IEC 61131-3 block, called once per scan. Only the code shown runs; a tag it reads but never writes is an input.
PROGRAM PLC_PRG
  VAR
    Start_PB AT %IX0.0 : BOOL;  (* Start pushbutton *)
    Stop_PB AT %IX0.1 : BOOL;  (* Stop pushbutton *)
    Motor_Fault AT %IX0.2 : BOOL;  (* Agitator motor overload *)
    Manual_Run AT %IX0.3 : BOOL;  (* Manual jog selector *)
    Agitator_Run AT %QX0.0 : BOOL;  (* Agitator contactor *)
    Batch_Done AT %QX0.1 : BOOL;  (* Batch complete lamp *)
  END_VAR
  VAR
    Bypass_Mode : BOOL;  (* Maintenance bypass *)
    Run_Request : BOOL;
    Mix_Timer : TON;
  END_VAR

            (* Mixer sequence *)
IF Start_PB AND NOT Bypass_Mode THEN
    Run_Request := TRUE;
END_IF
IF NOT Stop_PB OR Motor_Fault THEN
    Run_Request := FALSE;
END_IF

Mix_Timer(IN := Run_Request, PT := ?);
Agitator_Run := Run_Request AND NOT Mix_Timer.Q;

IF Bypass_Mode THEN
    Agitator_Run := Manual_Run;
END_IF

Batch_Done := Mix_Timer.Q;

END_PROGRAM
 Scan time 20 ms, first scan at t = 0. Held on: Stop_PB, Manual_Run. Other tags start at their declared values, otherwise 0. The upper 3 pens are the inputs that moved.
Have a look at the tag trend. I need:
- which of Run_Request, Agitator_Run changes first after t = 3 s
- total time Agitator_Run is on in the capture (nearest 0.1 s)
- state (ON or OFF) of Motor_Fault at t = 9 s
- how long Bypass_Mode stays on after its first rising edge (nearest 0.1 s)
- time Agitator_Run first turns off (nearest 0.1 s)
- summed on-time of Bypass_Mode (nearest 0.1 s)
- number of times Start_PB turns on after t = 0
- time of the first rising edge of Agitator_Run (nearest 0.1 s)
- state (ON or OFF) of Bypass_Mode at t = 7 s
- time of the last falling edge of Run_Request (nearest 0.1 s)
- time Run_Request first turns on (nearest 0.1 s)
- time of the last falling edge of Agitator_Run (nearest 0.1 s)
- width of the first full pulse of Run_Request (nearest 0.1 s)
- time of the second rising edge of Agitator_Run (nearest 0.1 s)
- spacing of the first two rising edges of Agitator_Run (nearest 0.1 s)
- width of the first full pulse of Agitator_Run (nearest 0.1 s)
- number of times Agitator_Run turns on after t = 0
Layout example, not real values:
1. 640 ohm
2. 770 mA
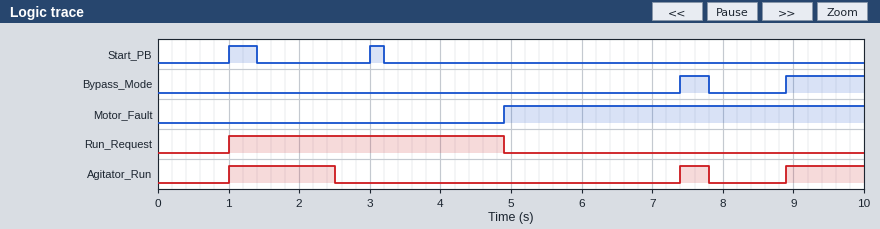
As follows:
1. Run_Request
2. 3.0 s
3. ON
4. 0.4 s
5. 2.5 s
6. 1.5 s
7. 2
8. 1.0 s
9. OFF
10. 4.9 s
11. 1.0 s
12. 7.8 s
13. 3.9 s
14. 7.4 s
15. 6.4 s
16. 1.5 s
17. 3
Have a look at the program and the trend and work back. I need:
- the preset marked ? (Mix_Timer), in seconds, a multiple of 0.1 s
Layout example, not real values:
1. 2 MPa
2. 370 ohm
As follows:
1. 1.5 s
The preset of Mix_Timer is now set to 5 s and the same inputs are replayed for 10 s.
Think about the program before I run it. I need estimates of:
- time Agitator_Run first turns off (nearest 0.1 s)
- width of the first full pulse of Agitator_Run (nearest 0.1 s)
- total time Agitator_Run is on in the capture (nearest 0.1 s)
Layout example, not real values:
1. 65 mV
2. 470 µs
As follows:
1. 4.9 s
2. 3.9 s
3. 5.4 s
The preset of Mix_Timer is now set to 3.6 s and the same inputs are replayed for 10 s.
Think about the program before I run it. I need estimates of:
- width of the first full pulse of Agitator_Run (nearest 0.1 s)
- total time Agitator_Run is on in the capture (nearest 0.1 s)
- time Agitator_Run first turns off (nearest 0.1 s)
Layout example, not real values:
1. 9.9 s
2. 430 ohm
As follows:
1. 3.6 s
2. 5.1 s
3. 4.6 s
